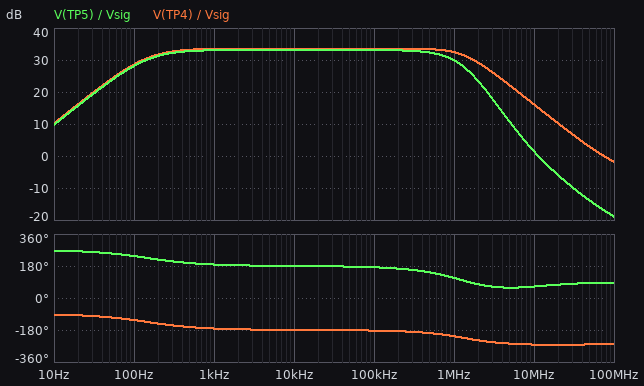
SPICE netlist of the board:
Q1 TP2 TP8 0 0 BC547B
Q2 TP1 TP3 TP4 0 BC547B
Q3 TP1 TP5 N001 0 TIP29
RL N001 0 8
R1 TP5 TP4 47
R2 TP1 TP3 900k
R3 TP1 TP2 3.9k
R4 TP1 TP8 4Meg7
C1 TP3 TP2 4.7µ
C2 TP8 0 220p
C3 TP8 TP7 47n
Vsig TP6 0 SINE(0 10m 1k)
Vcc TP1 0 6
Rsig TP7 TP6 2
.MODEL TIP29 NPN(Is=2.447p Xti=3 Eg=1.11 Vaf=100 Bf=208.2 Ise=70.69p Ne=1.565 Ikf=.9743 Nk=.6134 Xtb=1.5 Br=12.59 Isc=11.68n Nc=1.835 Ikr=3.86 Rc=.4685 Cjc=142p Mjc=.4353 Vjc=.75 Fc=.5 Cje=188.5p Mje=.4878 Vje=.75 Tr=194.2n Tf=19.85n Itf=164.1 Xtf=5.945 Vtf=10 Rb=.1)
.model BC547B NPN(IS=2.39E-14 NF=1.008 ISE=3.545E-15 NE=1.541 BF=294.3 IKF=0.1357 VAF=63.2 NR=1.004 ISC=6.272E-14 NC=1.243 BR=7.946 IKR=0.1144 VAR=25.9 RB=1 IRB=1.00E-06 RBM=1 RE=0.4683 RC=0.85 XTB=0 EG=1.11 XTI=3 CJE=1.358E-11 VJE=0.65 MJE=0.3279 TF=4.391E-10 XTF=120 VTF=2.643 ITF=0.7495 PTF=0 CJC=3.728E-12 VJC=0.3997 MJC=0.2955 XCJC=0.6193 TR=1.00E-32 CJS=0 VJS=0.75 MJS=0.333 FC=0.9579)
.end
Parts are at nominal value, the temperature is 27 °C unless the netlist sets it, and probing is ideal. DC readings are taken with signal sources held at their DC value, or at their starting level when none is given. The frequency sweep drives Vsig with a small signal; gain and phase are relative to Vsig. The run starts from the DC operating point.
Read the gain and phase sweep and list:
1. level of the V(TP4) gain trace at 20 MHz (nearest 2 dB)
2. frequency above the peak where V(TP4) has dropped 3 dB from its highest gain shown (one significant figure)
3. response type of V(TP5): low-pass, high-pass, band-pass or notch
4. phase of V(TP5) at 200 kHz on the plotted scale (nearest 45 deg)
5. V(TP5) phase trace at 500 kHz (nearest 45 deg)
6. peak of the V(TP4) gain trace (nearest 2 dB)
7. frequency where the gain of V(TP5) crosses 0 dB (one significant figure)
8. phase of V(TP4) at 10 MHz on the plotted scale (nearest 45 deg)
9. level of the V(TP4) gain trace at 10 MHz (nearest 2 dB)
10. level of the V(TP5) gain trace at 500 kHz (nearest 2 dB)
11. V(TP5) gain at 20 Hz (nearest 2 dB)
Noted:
10 dB
2 MHz
band-pass
180 deg
135 deg
34 dB
10 MHz
-270 deg
16 dB
32 dB
16 dB
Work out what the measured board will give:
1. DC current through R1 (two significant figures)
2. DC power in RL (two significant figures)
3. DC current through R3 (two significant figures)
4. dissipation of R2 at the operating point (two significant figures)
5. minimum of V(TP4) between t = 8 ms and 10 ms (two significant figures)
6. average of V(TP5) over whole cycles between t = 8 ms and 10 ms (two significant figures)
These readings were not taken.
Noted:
1.2 mA
130 mW
350 µA
15 µW
1.2 V
1.7 V
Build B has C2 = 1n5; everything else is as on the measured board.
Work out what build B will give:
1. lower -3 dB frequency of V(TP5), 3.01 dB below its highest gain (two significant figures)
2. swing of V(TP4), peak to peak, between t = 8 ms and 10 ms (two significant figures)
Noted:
140 Hz
910 mV
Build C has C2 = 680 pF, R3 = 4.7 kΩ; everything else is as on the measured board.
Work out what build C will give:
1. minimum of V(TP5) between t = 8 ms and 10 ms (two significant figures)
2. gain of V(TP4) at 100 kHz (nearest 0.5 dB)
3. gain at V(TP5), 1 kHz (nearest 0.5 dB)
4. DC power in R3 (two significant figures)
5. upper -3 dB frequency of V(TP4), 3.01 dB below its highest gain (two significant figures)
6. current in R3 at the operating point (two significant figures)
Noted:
1.1 V
35.0 dB
34.5 dB
560 µW
1.4 MHz
340 µA
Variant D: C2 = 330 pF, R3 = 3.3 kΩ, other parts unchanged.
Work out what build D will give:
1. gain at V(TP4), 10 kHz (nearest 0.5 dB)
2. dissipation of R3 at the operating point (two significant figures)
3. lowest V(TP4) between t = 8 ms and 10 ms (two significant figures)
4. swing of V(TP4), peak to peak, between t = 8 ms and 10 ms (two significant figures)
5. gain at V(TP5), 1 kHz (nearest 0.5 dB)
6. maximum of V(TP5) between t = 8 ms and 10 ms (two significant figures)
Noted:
32.0 dB
400 µW
1.3 V
790 mV
31.5 dB
2.0 V
